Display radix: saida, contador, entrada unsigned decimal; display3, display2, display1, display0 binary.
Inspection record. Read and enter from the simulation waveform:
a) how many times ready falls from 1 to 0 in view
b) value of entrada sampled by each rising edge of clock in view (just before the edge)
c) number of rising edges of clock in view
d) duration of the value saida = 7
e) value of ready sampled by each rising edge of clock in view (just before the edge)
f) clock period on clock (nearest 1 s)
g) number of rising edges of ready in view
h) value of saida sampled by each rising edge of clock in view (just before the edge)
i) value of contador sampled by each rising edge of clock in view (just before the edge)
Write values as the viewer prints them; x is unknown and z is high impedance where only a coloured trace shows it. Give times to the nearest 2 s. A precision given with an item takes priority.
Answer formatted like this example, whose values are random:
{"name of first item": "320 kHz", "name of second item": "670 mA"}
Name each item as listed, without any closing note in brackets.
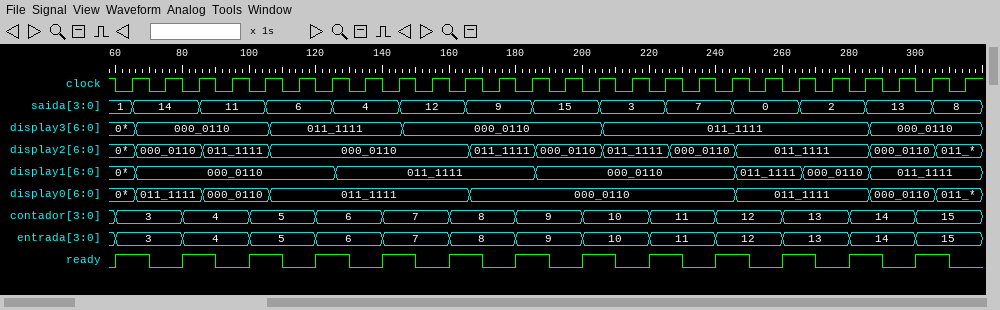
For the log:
{"how many times ready falls from 1 to 0 in view": "13", "value of entrada sampled by each rising edge of clock in view": "3, 3, 4, 4, 5, 5, 6, 6, 7, 7, 8, 8, 9, 9, 10, 10, 11, 11, 12, 12, 13, 13, 14, 14, 15, 15", "number of rising edges of clock in view": "26", "duration of the value saida = 7": "20 s", "value of ready sampled by each rising edge of clock in view": "1 0 1 0 1 0 1 0 1 0 1 0 1 0 1 0 1 0 1 0 1 0 1 0 1 0", "clock period on clock": "10 s", "number of rising edges of ready in view": "13", "value of saida sampled by each rising edge of clock in view": "1, 14, 14, 11, 11, 6, 6, 4, 4, 12, 12, 9, 9, 15, 15, 3, 3, 7, 7, 0, 0, 2, 2, 13, 13, 8", "value of contador sampled by each rising edge of clock in view": "3, 3, 4, 4, 5, 5, 6, 6, 7, 7, 8, 8, 9, 9, 10, 10, 11, 11, 12, 12, 13, 13, 14, 14, 15, 15"}
